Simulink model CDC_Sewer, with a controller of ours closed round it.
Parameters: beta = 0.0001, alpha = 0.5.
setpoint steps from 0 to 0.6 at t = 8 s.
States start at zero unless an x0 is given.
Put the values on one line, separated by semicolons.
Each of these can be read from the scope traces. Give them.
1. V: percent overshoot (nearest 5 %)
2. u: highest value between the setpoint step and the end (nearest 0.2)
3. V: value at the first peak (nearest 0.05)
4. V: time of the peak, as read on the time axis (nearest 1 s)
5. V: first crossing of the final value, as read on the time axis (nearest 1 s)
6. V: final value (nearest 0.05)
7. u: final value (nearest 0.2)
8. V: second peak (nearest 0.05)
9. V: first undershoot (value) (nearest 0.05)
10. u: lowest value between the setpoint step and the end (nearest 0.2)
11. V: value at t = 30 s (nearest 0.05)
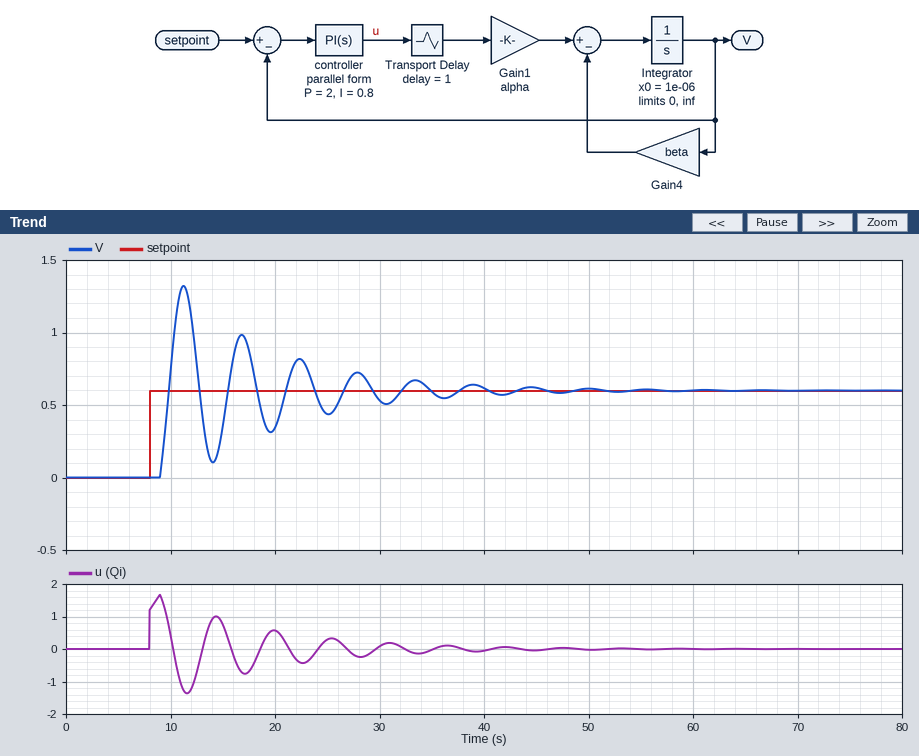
120 %; 1.6; 1.30; 11 s; 10 s; 0.60; 0.0; 1.00; 0.10; -1.4; 0.55
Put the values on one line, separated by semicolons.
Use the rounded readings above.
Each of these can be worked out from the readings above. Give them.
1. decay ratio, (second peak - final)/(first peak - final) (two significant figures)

0.57
